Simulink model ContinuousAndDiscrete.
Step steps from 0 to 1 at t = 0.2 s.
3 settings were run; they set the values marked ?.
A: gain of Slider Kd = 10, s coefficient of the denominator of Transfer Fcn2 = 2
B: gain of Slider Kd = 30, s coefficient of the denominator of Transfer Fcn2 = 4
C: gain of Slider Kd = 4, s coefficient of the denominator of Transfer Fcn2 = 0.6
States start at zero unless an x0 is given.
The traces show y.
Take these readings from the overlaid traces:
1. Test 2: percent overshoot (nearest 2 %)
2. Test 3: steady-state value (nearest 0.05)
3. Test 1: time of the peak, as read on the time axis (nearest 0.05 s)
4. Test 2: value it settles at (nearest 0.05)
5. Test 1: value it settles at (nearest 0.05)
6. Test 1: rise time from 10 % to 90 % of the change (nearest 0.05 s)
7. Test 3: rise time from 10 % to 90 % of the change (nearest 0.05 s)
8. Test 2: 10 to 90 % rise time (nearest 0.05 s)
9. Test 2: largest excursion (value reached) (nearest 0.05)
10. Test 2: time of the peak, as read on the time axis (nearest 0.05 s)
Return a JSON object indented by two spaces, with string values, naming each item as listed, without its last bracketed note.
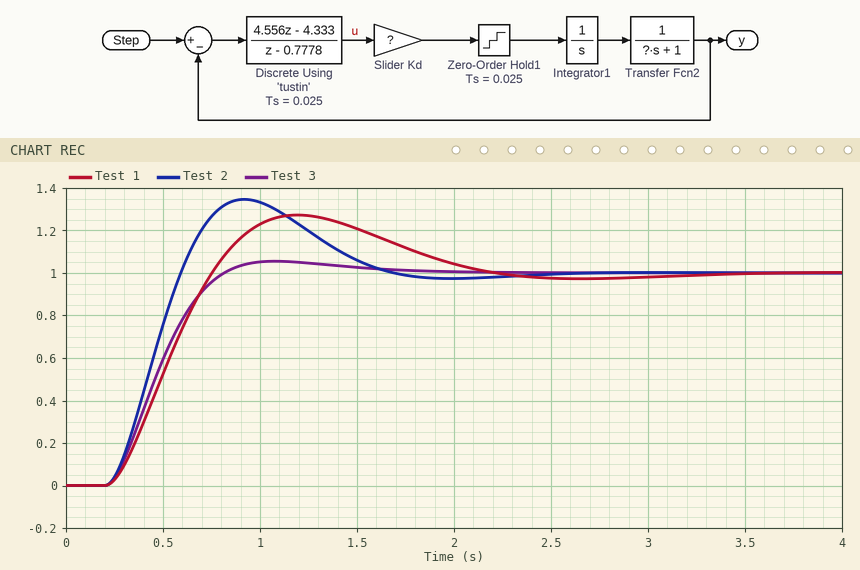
{
  "Test 2: percent overshoot": "34 %",
  "Test 3: steady-state value": "1.00",
  "Test 1: time of the peak, as read on the time axis": "1.20 s",
  "Test 2: value it settles at": "1.00",
  "Test 1: value it settles at": "1.00",
  "Test 1: rise time from 10 % to 90 % of the change": "0.40 s",
  "Test 3: rise time from 10 % to 90 % of the change": "0.40 s",
  "Test 2: 10 to 90 % rise time": "0.25 s",
  "Test 2: largest excursion (value reached)": "1.35",
  "Test 2: time of the peak, as read on the time axis": "0.90 s"
}
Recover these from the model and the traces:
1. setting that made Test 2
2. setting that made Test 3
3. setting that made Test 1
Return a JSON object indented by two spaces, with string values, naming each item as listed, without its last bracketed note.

{
  "setting that made Test 2": "B",
  "setting that made Test 3": "C",
  "setting that made Test 1": "A"
}
